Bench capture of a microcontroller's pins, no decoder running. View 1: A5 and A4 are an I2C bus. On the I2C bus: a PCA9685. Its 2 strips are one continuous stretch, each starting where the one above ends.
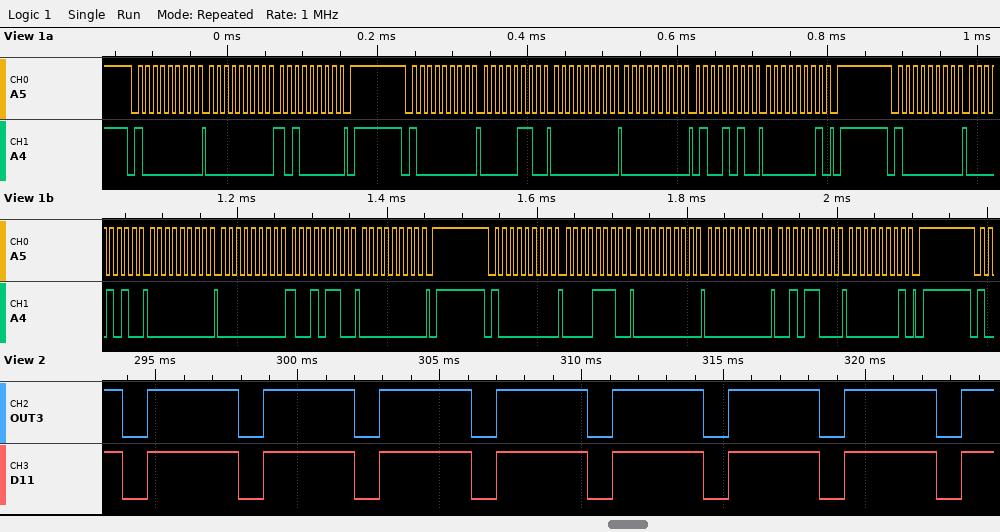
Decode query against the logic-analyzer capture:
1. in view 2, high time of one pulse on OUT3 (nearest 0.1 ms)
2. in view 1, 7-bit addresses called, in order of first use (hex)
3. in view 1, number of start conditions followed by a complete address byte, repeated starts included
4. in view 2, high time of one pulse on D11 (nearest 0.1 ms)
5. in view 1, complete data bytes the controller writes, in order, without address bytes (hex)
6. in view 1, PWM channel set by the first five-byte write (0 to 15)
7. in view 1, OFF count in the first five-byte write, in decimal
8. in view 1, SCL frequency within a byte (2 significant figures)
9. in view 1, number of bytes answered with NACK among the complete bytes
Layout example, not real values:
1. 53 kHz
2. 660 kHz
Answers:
1. 3.2 ms
2. 0x40
3. 4
4. 3.2 ms
5. 00 A0 06 00 00 4A 01 0A 00 00 96 00 0E 00 00 2C 01
6. 0
7. 330
8. 100 kHz
9. 0
